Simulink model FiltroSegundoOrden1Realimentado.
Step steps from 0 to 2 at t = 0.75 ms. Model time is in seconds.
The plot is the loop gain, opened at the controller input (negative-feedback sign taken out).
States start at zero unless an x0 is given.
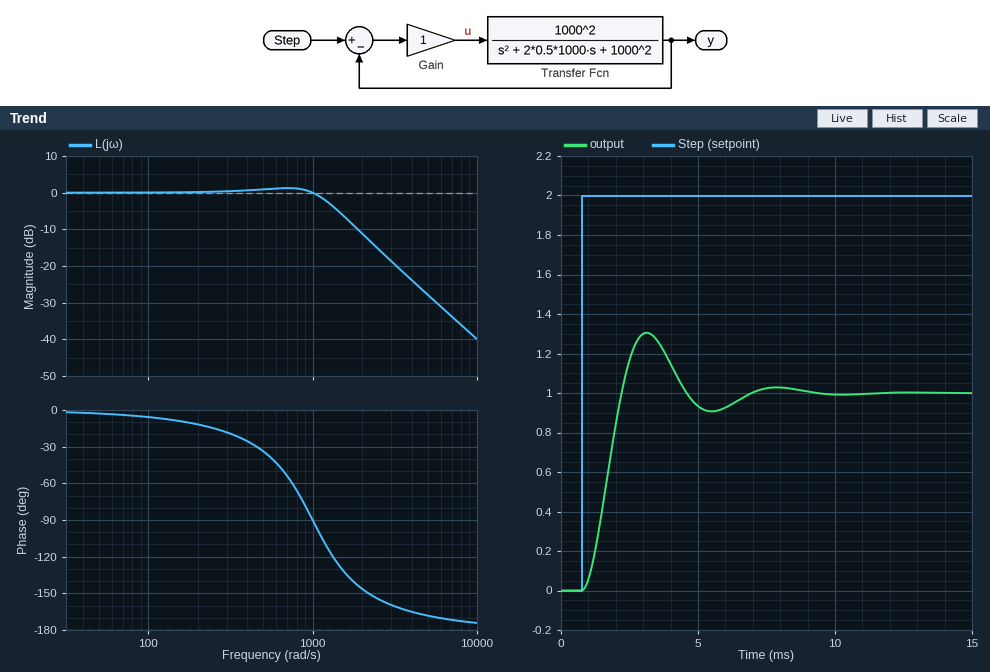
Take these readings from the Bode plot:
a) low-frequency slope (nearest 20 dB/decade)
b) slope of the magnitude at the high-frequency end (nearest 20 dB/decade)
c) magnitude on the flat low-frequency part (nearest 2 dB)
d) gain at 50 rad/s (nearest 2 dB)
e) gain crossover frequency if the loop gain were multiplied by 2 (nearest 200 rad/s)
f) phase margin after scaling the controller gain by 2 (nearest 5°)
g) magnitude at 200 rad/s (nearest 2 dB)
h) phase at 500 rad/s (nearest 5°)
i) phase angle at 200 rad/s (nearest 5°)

0 dB/decade
-40 dB/decade
0 dB
0 dB
1600 rad/s
50°
0 dB
-35°
-10°
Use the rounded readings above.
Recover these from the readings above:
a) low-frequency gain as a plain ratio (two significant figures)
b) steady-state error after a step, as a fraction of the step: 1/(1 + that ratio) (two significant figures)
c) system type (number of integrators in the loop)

1.0
0.50
0
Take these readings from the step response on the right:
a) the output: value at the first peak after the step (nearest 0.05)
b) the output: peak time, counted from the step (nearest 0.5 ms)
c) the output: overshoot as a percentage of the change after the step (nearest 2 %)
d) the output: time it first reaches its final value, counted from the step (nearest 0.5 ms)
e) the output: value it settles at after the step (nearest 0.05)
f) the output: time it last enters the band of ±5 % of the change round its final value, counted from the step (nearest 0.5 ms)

1.30
2.5 ms
30 %
1.5 ms
1.00
5.5 ms
